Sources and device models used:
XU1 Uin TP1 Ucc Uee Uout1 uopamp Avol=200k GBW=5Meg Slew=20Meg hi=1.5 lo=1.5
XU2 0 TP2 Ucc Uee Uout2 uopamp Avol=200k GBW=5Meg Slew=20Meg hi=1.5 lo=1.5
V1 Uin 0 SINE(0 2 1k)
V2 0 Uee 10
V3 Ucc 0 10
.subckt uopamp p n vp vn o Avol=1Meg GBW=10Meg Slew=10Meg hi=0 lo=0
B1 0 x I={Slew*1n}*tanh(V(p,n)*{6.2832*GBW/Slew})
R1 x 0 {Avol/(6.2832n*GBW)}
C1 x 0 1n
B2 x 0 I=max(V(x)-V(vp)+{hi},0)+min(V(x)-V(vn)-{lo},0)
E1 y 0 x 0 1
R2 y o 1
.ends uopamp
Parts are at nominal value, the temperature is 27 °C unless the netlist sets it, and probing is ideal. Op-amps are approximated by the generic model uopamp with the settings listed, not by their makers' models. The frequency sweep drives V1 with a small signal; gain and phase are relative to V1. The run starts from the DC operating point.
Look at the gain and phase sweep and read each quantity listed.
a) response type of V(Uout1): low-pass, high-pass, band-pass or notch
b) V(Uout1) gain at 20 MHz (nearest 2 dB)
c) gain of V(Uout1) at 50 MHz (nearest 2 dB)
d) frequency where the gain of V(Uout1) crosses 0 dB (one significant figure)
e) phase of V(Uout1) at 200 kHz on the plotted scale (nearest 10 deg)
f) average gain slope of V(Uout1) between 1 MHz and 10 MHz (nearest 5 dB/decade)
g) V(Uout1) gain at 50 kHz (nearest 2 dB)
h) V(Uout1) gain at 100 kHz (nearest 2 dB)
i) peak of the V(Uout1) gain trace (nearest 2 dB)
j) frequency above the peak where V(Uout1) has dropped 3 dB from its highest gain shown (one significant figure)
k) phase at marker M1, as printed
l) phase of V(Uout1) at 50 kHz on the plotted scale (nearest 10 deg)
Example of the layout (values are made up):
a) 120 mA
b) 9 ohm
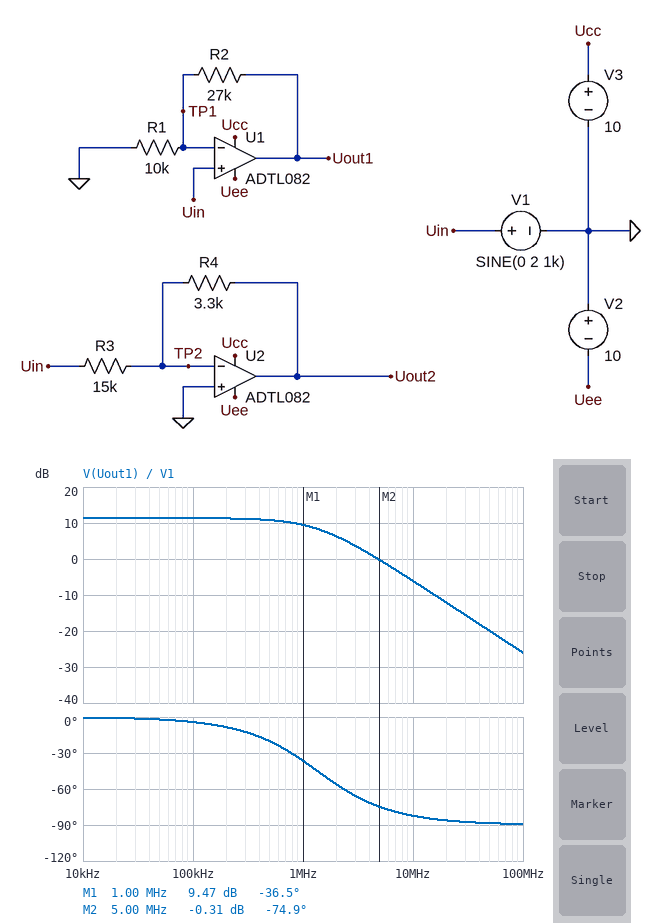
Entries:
a) low-pass
b) -12 dB
c) -20 dB
d) 5 MHz
e) -10 deg
f) -15 dB/decade
g) 12 dB
h) 12 dB
i) 12 dB
j) 1 MHz
k) -36.5 deg
l) 0 deg
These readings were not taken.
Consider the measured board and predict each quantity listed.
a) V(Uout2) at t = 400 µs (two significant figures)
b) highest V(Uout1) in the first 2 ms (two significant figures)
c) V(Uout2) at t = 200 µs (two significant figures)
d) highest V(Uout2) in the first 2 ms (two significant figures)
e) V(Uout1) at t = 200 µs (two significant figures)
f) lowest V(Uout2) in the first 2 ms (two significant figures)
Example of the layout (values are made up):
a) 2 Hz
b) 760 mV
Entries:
a) -260 mV
b) 7.4 V
c) -420 mV
d) 440 mV
e) 7.0 V
f) -440 mV
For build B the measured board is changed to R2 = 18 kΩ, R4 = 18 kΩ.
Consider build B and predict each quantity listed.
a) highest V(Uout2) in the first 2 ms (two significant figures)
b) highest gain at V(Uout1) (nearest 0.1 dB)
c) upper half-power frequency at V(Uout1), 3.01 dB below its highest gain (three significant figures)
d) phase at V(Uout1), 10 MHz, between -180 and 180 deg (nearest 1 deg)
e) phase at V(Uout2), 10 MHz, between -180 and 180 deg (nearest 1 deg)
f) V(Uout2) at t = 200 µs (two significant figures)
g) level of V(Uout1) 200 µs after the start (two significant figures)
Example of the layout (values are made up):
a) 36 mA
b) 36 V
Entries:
a) 2.4 V
b) 8.9 dB
c) 1.79 MHz
d) -80 deg
e) 103 deg
f) -2.3 V
g) 5.3 V
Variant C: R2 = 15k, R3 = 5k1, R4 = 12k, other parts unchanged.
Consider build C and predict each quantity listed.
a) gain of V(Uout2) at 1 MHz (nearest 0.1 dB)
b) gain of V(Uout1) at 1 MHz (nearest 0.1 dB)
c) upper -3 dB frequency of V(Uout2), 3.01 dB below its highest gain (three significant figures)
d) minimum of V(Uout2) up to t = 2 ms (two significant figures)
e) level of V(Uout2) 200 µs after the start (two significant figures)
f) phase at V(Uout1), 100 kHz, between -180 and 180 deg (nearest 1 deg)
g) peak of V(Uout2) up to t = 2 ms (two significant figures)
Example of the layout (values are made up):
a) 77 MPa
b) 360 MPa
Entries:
a) 5.8 dB
b) 7.0 dB
c) 1.49 MHz
d) -4.7 V
e) -4.5 V
f) -3 deg
g) 4.7 V
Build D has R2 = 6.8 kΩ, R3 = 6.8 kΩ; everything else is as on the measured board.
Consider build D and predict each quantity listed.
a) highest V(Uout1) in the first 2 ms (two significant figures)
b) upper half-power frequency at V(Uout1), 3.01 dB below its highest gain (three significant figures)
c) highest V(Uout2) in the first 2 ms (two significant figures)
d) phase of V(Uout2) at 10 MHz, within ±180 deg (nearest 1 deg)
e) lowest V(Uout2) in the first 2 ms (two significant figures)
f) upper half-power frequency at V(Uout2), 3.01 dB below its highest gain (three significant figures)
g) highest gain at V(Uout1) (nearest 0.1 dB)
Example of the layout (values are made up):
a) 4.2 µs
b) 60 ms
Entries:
a) 3.4 V
b) 2.98 MHz
c) 970 mV
d) 109 deg
e) -970 mV
f) 3.37 MHz
g) 4.5 dB
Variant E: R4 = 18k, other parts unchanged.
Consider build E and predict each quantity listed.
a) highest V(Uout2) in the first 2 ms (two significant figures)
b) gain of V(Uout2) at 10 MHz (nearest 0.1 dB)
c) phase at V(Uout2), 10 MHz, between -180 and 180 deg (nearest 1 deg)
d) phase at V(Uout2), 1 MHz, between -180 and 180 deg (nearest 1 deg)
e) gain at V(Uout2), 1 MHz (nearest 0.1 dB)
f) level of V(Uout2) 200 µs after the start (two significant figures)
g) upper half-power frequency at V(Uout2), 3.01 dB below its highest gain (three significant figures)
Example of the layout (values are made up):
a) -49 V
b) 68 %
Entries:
a) 2.4 V
b) -11.5 dB
c) 103 deg
d) 156 deg
e) 0.8 dB
f) -2.3 V
g) 2.27 MHz
